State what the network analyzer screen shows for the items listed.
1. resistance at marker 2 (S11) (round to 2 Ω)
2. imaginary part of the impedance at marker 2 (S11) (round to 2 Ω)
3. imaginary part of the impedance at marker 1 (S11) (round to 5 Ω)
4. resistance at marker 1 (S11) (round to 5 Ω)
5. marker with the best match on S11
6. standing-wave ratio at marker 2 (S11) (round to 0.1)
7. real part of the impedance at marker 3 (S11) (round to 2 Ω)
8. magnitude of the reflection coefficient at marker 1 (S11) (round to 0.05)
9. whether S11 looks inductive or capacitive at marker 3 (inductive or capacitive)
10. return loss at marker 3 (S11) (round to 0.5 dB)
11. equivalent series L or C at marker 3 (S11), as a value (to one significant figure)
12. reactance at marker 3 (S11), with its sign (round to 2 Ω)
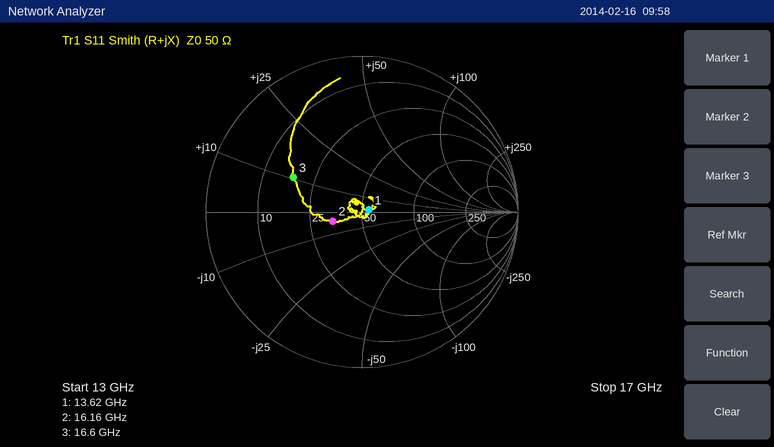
34 Ω
-4 Ω
0 Ω
55 Ω
marker 1
1.5
18 Ω
0.05
inductive
6.0 dB
100 pH
+10 Ω
